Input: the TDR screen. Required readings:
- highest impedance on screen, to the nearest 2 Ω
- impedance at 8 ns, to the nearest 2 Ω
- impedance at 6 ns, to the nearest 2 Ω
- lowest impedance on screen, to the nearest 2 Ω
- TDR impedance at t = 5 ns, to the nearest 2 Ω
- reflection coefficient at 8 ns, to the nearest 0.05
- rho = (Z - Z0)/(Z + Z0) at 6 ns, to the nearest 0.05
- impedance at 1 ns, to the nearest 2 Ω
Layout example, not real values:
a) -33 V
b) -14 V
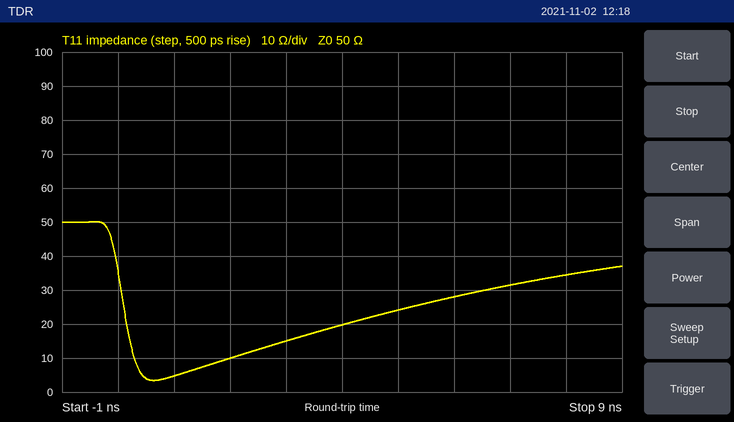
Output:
a) 50 Ω
b) 34 Ω
c) 28 Ω
d) 4 Ω
e) 24 Ω
f) -0.20
g) -0.30
h) 4 Ω
